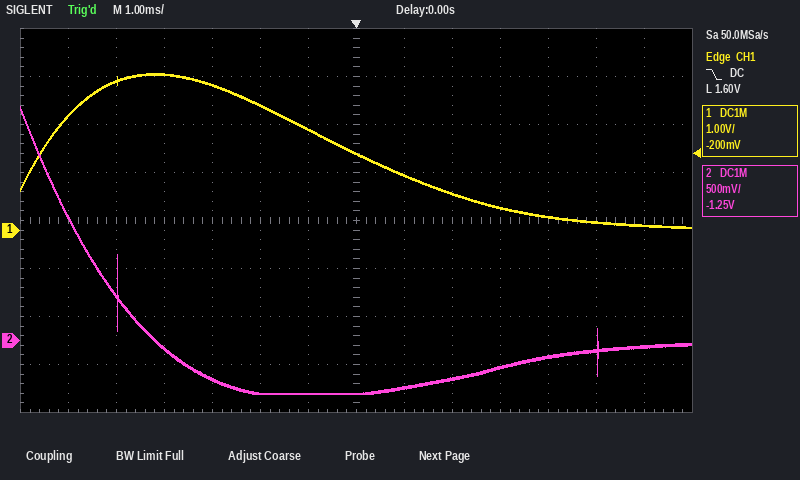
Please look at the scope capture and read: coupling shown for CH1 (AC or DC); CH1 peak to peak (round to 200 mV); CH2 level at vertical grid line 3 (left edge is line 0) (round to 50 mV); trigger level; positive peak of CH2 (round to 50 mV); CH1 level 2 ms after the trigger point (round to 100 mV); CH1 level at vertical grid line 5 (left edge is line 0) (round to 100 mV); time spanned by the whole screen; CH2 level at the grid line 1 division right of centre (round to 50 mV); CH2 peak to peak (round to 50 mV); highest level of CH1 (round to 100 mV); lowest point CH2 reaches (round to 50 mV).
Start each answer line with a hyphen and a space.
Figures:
- DC
- 3.2 V
- -100 mV
- 1.60 V
- 2.45 V
- 800 mV
- 2.6 V
- 14 ms
- -500 mV
- 3.00 V
- 3.3 V
- -550 mV
